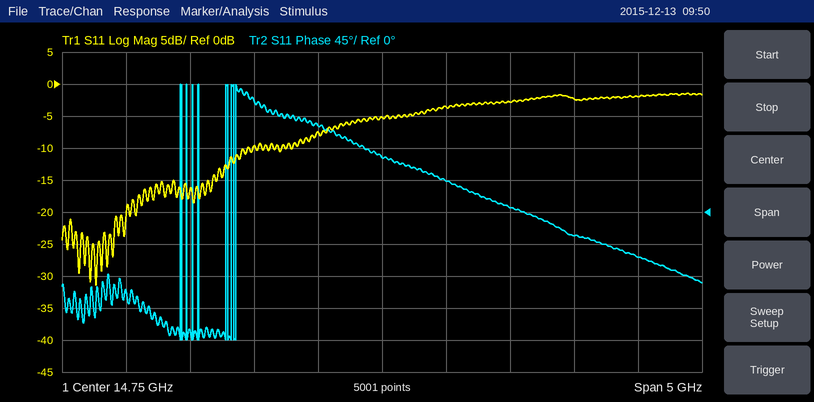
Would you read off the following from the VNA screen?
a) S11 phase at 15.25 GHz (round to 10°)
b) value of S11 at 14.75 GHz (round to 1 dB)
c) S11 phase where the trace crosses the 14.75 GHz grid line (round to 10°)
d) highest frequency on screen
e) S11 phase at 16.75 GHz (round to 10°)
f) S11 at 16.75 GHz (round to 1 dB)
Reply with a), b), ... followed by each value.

a) 40°
b) -5 dB
c) 80°
d) 17.25 GHz
e) -60°
f) -2 dB
